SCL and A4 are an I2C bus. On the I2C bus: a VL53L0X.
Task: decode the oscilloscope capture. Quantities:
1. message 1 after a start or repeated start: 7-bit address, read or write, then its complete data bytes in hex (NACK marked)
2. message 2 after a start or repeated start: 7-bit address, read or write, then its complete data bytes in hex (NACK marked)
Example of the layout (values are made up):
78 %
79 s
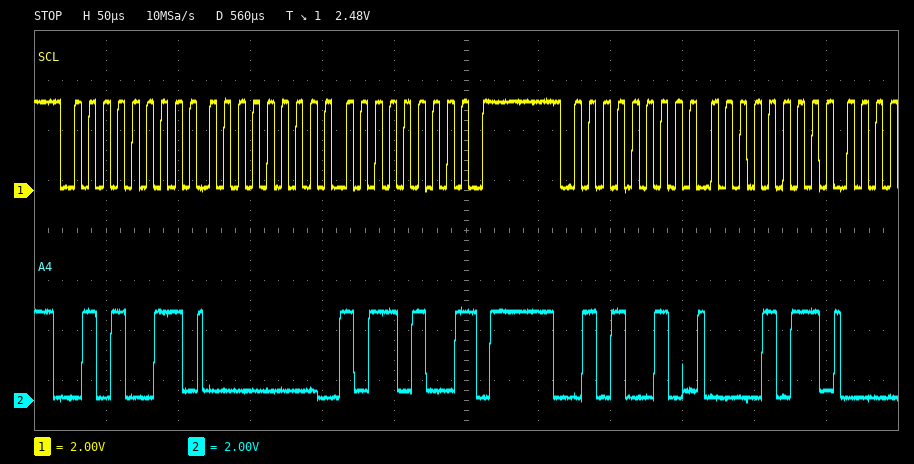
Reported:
0x29 read: 00 B4 NACK
0x29 write: 0B
